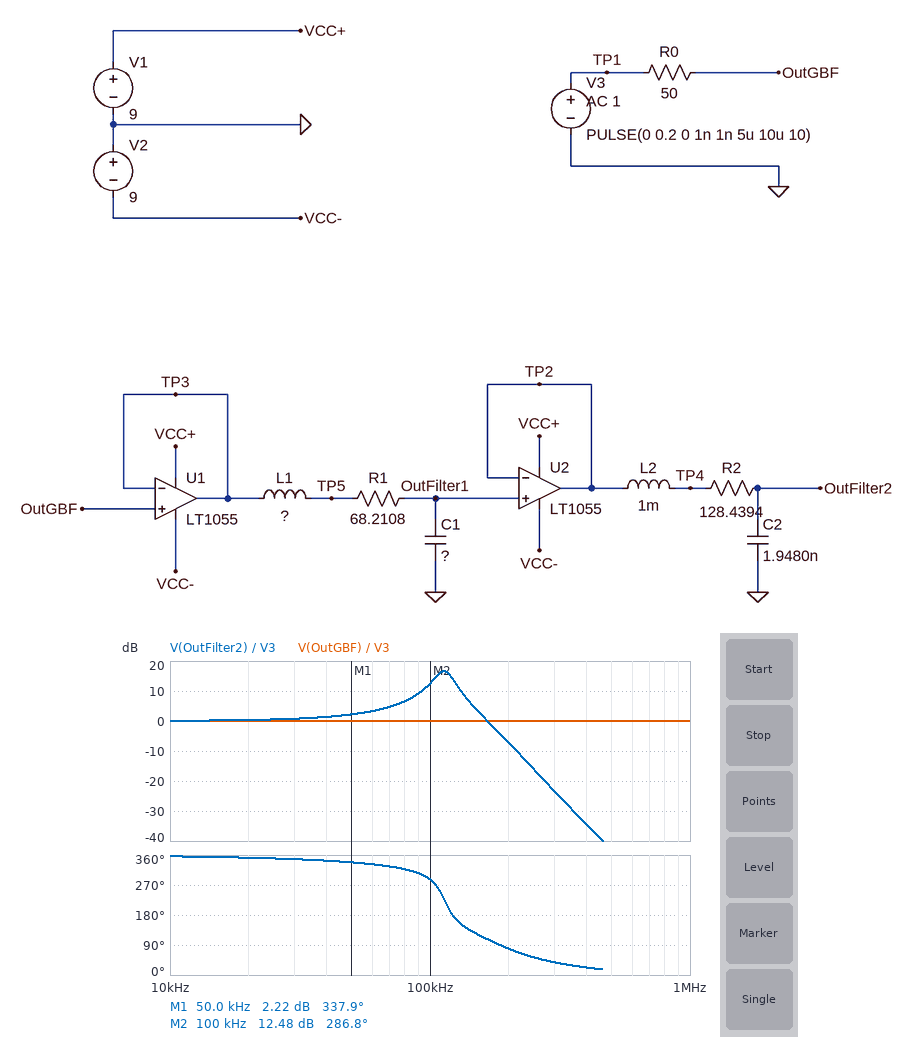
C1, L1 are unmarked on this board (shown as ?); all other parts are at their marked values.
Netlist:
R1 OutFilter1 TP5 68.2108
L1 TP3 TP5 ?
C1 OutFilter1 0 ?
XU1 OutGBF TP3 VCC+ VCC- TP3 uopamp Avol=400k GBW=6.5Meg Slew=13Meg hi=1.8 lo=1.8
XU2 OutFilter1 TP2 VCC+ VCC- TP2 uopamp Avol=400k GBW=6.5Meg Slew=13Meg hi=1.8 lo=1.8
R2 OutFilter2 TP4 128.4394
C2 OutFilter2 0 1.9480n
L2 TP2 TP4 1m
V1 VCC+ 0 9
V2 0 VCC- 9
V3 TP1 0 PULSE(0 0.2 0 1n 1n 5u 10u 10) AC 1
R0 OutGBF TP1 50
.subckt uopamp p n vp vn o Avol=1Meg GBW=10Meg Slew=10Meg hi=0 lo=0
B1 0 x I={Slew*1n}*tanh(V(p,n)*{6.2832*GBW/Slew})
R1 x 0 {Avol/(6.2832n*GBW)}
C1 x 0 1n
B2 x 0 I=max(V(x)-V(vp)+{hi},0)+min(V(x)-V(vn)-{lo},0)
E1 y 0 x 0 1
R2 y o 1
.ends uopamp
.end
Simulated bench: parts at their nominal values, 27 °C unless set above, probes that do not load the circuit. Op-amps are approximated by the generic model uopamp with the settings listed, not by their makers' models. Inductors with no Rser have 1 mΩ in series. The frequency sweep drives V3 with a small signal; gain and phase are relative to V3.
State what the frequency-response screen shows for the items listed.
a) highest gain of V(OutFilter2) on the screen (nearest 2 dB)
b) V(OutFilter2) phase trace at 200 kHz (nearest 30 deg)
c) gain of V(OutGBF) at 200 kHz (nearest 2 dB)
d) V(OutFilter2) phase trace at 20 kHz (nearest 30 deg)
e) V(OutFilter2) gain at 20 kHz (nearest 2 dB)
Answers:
16 dB
90 deg
0 dB
360 deg
0 dB
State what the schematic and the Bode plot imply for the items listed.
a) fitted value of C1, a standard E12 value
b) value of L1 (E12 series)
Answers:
12 nF
68 µH
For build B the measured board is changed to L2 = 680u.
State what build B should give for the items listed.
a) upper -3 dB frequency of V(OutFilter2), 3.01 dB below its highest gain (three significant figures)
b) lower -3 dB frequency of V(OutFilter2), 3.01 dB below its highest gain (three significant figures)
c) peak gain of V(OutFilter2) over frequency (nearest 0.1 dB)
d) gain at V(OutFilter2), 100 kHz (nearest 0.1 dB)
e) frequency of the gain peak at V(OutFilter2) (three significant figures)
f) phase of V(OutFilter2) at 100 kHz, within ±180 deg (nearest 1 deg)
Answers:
151 kHz
121 kHz
15.2 dB
7.4 dB
137 kHz
-57 deg
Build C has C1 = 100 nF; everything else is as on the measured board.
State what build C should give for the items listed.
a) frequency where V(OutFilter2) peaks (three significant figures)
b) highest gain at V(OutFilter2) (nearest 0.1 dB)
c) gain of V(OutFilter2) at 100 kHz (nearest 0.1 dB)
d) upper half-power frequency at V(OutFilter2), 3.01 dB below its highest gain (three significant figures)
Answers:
112 kHz
0.3 dB
-2.2 dB
121 kHz
